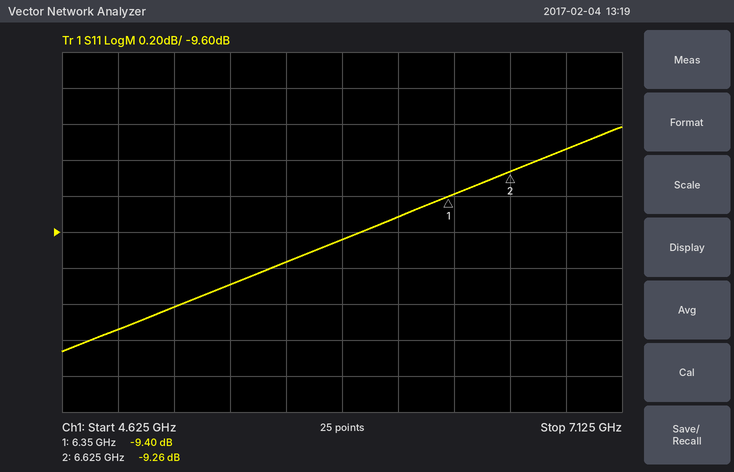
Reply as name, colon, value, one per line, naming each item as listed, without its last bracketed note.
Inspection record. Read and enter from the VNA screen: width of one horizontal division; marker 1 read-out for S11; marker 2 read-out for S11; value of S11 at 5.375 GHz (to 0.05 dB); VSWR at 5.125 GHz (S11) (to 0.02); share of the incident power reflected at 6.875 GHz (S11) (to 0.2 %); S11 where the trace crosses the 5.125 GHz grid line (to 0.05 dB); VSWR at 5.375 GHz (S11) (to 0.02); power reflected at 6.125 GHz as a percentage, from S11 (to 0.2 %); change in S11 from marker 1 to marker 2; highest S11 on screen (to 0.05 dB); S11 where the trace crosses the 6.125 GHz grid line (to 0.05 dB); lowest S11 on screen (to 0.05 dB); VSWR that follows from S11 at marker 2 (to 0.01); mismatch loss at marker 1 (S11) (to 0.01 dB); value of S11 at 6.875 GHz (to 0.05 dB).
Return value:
width of one horizontal division: 250 MHz
marker 1 read-out for S11: -9.40 dB
marker 2 read-out for S11: -9.26 dB
value of S11 at 5.375 GHz: -9.90 dB
VSWR at 5.125 GHz (S11): 1.92
share of the incident power reflected at 6.875 GHz (S11): 12.2 %
S11 where the trace crosses the 5.125 GHz grid line: -10.00 dB
VSWR at 5.375 GHz (S11): 1.94
power reflected at 6.125 GHz as a percentage, from S11: 11.2 %
change in S11 from marker 1 to marker 2: 0.14 dB
highest S11 on screen: -9.00 dB
S11 where the trace crosses the 6.125 GHz grid line: -9.50 dB
lowest S11 on screen: -10.25 dB
VSWR that follows from S11 at marker 2: 2.05
mismatch loss at marker 1 (S11): 0.53 dB
value of S11 at 6.875 GHz: -9.15 dB
